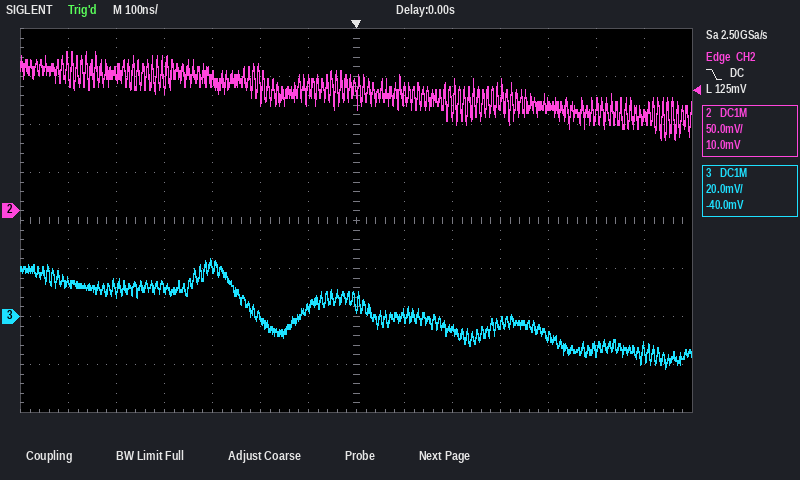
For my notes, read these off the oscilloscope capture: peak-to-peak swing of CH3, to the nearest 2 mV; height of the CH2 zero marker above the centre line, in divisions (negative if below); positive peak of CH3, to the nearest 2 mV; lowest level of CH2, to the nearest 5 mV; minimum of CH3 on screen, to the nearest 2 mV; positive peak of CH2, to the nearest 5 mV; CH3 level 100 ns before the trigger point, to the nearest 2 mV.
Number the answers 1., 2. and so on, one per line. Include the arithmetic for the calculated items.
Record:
1. 24 mV − (-22 mV) = 46 mV
2. +0.2 div
3. 24 mV
4. 75 mV
5. -22 mV
6. 165 mV
7. 4 mV
